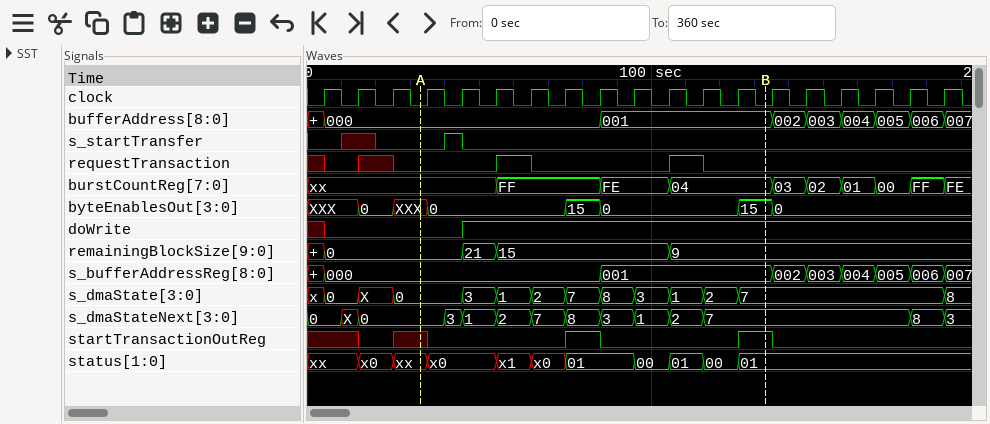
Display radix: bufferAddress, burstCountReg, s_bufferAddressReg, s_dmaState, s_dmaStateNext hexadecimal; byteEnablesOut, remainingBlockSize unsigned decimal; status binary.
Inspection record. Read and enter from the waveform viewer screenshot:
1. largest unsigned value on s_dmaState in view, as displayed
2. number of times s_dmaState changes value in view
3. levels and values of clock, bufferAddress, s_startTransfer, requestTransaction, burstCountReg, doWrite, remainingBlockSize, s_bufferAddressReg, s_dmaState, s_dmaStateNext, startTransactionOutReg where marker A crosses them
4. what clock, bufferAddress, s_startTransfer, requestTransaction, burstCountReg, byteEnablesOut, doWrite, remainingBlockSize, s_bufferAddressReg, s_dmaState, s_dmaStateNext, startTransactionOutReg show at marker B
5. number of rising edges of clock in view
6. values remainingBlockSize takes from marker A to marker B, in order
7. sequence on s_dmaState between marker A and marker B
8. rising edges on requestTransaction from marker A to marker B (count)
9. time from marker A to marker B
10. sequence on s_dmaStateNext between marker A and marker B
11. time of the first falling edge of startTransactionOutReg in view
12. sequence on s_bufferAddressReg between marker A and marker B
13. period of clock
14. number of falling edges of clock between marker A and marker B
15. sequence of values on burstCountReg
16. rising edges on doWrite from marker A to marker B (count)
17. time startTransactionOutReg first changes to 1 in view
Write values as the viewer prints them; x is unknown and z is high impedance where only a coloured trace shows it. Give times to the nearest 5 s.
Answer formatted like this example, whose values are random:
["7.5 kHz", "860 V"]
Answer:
["8", "13", "clock=0, bufferAddress=000, s_startTransfer=0, requestTransaction=0, burstCountReg=xx, doWrite=0, remainingBlockSize=0, s_bufferAddressReg=000, s_dmaState=0, s_dmaStateNext=0, startTransactionOutReg=x", "clock=0, bufferAddress=001, s_startTransfer=0, requestTransaction=0, burstCountReg=04, byteEnablesOut=15, doWrite=1, remainingBlockSize=9, s_bufferAddressReg=001, s_dmaState=7, s_dmaStateNext=7, startTransactionOutReg=1", "19", "0, 21, 15, 9", "0, 3, 1, 2, 7, 8, 3, 1, 2, 7", "2", "100 s", "0, 3, 1, 2, 7, 8, 3, 1, 2, 7", "85 s", "000, 001", "10 s", "10", "xx, FF, FE, 04, 03, 02, 01, 00, FF, FE", "1", "75 s"]
